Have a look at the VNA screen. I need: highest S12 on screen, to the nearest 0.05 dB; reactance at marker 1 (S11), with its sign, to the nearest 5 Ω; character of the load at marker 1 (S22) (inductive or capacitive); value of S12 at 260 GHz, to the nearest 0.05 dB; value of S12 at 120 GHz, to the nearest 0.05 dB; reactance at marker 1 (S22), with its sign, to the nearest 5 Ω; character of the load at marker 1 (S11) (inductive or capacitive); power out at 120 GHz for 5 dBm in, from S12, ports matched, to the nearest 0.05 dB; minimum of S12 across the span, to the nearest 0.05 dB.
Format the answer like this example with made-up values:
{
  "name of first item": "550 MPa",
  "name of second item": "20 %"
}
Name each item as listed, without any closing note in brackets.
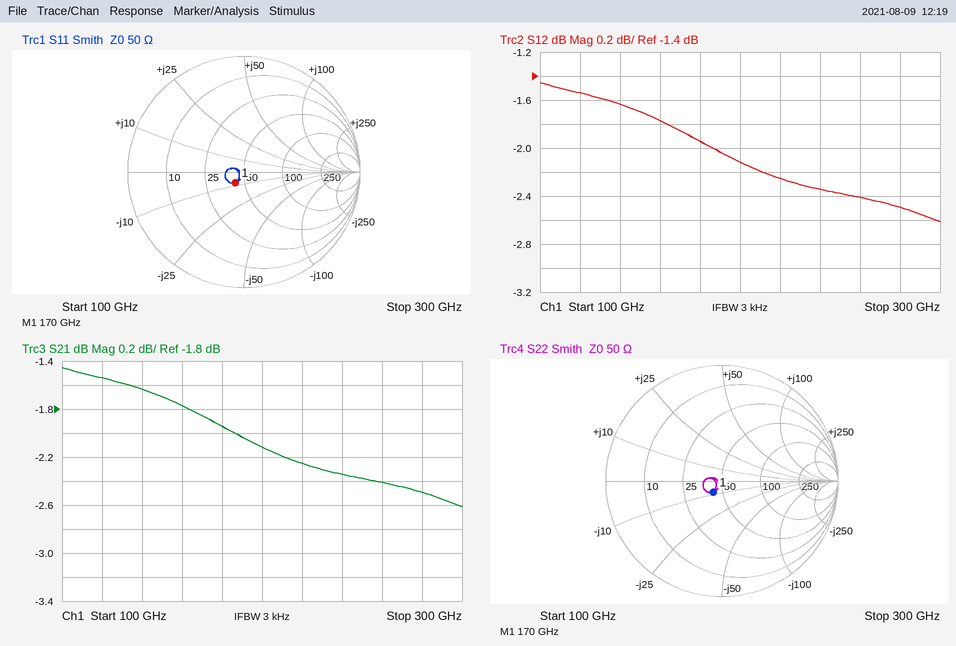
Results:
{
  "highest S12 on screen, to the nearest 0.05 dB": "-1.45 dB",
  "reactance at marker 1 (S11), with its sign, to the nearest 5 Ω": "-10 Ω",
  "character of the load at marker 1 (S22)": "capacitive",
  "value of S12 at 260 GHz, to the nearest 0.05 dB": "-2.40 dB",
  "value of S12 at 120 GHz, to the nearest 0.05 dB": "-1.55 dB",
  "reactance at marker 1 (S22), with its sign, to the nearest 5 Ω": "-10 Ω",
  "character of the load at marker 1 (S11)": "capacitive",
  "power out at 120 GHz for 5 dBm in, from S12, ports matched, to the nearest 0.05 dB": "3.45 dBm",
  "minimum of S12 across the span, to the nearest 0.05 dB": "-2.60 dB"
}
